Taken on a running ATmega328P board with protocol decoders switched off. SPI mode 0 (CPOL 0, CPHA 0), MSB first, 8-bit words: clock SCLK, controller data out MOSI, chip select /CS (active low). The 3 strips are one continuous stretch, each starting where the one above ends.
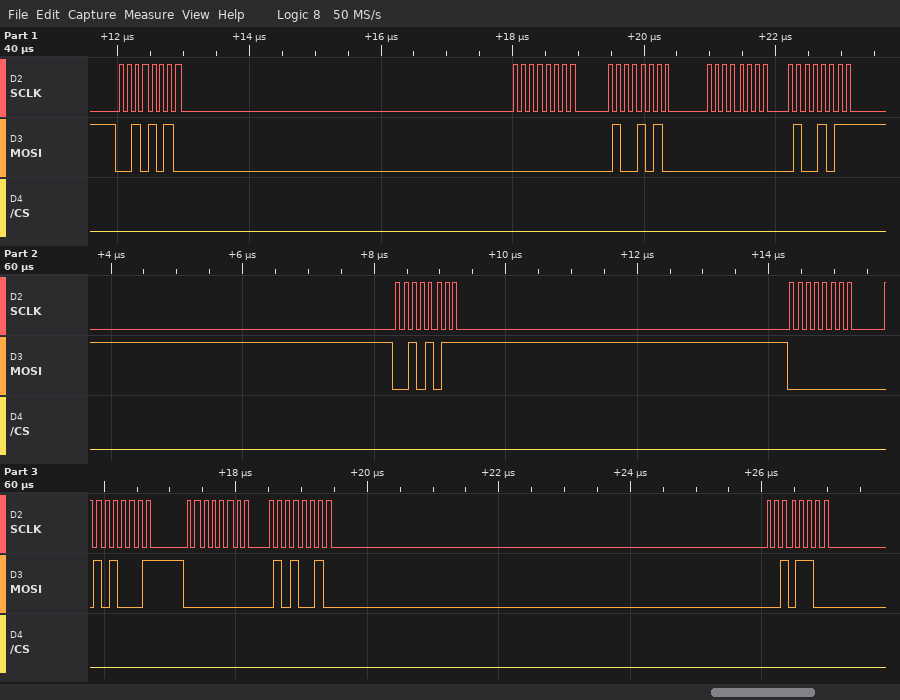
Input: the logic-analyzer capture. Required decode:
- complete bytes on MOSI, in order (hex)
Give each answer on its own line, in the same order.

2A 00 4A 00 4B 2B 00 51 00 52 2C
